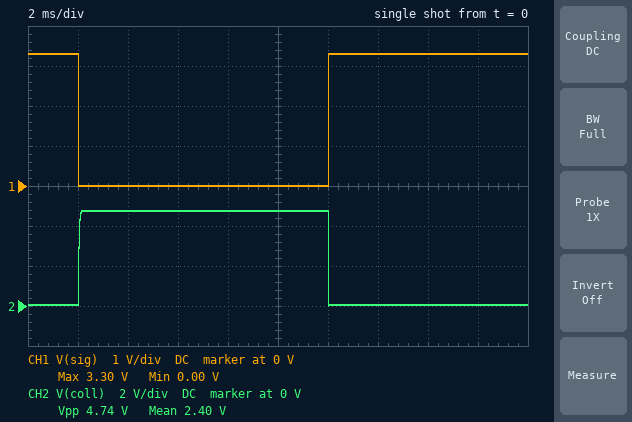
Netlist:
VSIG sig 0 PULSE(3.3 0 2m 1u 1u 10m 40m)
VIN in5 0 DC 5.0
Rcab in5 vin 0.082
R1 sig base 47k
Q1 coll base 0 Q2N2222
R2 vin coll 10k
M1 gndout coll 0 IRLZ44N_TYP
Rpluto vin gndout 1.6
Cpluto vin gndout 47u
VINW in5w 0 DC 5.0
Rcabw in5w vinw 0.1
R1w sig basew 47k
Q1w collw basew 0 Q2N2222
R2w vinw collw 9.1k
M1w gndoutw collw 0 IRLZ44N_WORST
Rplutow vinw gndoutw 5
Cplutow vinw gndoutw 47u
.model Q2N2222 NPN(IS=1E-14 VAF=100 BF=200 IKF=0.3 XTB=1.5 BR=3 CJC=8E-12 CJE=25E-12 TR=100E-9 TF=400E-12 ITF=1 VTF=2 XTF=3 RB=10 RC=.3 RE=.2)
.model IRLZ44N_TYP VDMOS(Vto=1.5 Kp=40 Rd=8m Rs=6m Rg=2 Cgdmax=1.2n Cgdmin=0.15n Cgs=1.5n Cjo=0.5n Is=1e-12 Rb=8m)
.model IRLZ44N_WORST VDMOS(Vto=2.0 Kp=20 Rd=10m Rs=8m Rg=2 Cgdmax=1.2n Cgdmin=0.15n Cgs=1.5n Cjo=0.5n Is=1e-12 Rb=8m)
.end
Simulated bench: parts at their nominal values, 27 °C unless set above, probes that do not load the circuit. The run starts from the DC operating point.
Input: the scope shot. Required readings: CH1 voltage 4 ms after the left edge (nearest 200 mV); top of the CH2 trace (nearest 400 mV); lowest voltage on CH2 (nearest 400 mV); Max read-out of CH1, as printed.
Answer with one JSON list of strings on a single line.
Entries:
["0 V", "4.8 V", "0 V", "3.30 V"]
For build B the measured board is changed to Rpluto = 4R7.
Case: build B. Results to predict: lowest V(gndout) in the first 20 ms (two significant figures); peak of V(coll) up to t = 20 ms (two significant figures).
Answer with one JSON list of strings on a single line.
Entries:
["22 mV", "4.9 V"]
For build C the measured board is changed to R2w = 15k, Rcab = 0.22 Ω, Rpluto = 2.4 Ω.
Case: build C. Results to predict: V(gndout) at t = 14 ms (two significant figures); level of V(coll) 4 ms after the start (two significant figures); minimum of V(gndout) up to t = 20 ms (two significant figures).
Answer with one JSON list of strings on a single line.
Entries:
["5.0 V", "4.6 V", "42 mV"]
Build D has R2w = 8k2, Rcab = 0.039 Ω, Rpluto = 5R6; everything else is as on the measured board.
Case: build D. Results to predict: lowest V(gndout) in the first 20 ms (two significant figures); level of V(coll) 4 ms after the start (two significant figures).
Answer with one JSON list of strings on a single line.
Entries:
["19 mV", "5.0 V"]
